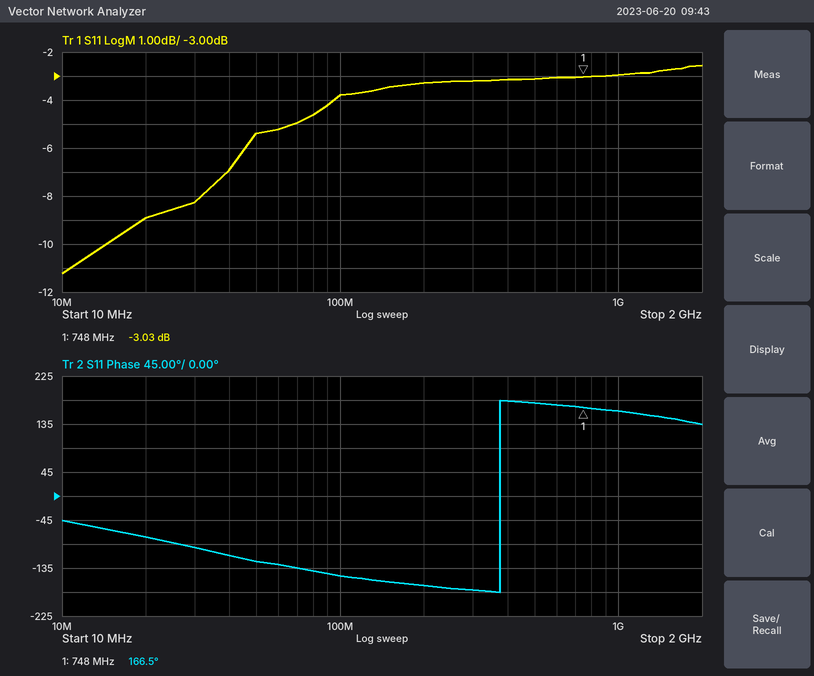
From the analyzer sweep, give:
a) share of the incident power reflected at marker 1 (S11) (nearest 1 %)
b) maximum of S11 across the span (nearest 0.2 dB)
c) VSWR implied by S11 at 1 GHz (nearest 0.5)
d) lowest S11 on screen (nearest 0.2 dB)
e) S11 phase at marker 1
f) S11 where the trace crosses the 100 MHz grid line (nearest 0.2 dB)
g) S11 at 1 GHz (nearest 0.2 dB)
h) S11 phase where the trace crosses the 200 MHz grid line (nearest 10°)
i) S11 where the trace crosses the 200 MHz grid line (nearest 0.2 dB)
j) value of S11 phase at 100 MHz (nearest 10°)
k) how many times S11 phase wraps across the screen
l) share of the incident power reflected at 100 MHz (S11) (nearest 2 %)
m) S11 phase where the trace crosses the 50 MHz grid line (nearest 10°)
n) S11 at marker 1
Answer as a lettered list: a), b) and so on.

a) 50 %
b) -2.6 dB
c) 6.0
d) -11.2 dB
e) 166.5°
f) -3.8 dB
g) -3.0 dB
h) -170°
i) -3.2 dB
j) -150°
k) 1
l) 42 %
m) -120°
n) -3.03 dB
